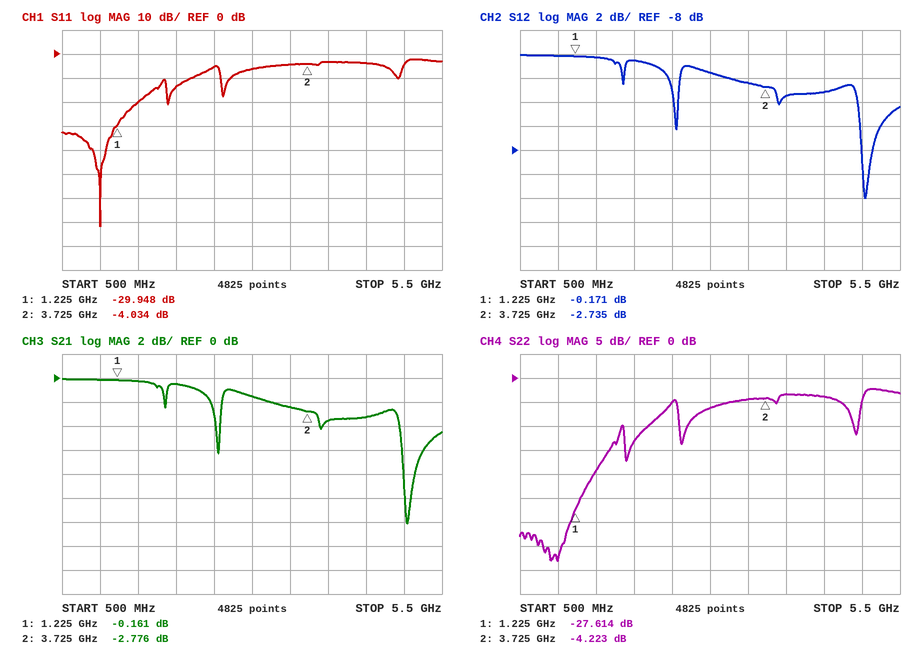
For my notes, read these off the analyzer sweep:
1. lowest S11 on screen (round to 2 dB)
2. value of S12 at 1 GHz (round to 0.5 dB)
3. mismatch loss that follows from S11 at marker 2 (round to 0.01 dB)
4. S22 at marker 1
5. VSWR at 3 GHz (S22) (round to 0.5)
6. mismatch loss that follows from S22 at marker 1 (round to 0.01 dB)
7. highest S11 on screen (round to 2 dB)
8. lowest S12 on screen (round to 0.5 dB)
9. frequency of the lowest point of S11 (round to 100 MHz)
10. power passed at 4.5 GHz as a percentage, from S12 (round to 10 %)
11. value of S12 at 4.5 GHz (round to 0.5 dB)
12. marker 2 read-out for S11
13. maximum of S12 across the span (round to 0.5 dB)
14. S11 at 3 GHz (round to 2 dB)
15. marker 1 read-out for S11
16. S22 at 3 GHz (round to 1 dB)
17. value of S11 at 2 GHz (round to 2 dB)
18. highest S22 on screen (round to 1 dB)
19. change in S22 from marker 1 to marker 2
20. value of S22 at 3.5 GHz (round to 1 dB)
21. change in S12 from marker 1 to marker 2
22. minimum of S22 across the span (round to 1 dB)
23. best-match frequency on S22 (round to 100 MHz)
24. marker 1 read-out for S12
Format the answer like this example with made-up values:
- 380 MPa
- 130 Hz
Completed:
- -72 dB
- 0.0 dB
- 2.18 dB
- -27.614 dB
- 3.0
- 0.01 dB
- -2 dB
- -12.0 dB
- 1.0 GHz
- 50 %
- -3.0 dB
- -4.034 dB
- 0.0 dB
- -6 dB
- -29.948 dB
- -6 dB
- -14 dB
- -2 dB
- 23.391 dB
- -4 dB
- -2.564 dB
- -38 dB
- 1.0 GHz
- -0.171 dB
